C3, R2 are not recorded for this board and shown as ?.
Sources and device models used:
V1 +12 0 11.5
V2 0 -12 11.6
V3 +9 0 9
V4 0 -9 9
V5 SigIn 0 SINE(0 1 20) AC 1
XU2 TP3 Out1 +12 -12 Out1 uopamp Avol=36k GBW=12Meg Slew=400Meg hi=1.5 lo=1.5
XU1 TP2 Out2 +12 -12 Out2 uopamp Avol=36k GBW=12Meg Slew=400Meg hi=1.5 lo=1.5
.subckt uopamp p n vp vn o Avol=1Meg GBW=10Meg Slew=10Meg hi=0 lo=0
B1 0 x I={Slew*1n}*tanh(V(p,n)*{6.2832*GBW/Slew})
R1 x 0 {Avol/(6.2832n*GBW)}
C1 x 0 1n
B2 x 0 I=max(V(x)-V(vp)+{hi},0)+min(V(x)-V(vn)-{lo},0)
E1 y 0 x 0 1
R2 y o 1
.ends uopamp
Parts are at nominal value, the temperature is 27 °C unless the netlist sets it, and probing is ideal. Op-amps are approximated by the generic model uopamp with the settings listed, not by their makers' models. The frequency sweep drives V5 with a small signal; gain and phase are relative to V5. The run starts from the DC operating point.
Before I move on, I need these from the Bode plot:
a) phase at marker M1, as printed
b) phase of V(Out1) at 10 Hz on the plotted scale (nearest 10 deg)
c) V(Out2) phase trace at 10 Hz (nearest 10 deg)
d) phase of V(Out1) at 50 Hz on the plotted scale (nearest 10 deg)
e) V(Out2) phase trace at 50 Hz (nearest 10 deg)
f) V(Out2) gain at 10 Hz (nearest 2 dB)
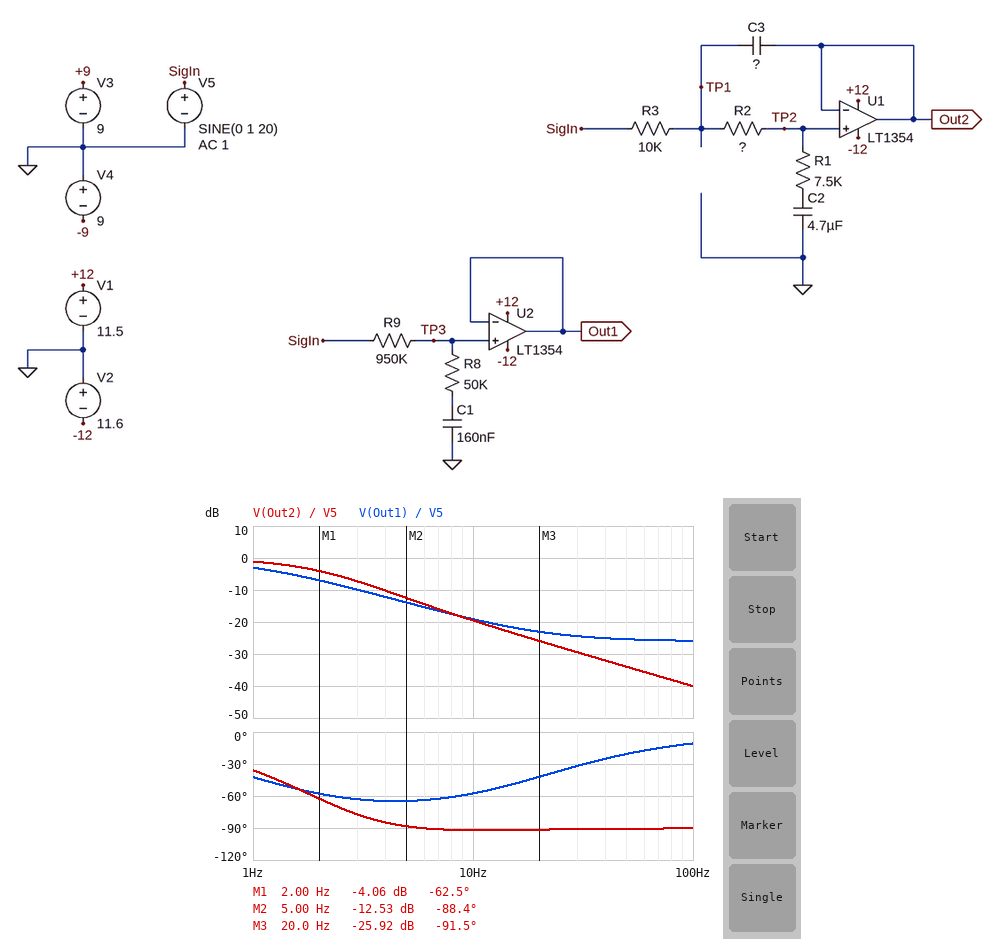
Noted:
-62.5 deg
-60 deg
-90 deg
-20 deg
-90 deg
-20 dB
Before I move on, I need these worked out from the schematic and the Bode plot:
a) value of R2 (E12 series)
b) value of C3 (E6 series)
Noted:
12 kΩ
10 µF
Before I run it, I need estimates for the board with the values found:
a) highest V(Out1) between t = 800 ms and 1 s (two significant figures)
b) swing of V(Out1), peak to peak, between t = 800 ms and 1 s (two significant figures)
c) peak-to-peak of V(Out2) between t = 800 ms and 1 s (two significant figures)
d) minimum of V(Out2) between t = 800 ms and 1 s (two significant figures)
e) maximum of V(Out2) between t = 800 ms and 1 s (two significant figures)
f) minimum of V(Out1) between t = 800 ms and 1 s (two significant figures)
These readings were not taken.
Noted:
71 mV
140 mV
100 mV
-51 mV
51 mV
-70 mV
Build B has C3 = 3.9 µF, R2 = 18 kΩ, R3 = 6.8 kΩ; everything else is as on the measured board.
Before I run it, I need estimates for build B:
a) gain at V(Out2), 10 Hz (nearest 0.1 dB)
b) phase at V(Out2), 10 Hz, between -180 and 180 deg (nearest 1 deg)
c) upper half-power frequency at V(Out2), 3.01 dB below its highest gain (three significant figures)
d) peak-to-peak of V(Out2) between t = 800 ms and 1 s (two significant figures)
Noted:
-14.1 dB
-64 deg
1.24 Hz
230 mV
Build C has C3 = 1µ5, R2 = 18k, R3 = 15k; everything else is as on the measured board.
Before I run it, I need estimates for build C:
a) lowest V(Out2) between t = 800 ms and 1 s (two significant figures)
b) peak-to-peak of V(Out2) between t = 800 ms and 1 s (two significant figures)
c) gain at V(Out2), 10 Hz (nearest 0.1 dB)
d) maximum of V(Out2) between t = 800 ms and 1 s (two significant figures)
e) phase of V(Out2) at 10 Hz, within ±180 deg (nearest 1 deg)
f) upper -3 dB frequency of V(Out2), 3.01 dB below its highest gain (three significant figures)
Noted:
-120 mV
240 mV
-15.0 dB
120 mV
-53 deg
918 mHz
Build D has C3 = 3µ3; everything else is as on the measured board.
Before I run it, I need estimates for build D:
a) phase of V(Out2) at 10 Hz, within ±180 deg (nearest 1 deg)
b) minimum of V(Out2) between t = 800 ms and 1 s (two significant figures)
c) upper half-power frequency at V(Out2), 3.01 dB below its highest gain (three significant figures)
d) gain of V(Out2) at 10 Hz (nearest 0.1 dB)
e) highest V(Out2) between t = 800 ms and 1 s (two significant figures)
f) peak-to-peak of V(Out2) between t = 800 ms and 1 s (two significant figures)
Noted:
-60 deg
-140 mV
1.38 Hz
-12.9 dB
140 mV
270 mV
